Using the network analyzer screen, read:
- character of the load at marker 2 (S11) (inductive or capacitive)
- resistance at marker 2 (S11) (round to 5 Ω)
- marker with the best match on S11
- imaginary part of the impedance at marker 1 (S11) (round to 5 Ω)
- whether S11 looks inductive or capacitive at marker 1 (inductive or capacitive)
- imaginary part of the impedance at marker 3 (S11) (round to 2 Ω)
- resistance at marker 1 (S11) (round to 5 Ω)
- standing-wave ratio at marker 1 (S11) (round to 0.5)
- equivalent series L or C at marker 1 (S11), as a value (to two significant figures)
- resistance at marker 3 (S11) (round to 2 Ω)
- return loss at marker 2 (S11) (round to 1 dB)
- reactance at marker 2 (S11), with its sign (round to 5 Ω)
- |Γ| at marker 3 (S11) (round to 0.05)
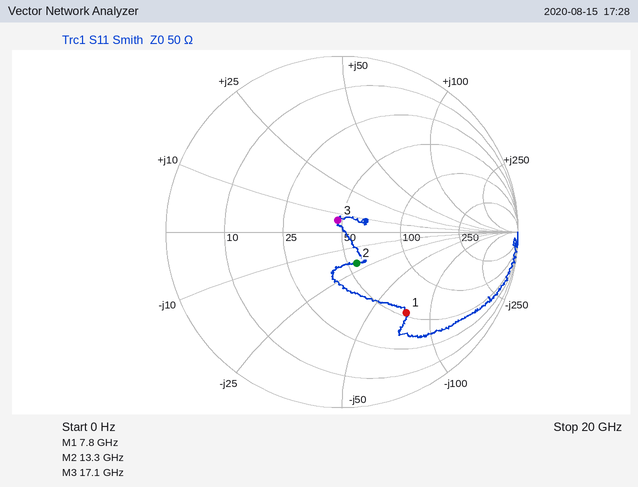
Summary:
capacitive
55 Ω
marker 3
-75 Ω
capacitive
+6 Ω
55 Ω
4.0
270 fF
48 Ω
14 dB
-20 Ω
0.05
